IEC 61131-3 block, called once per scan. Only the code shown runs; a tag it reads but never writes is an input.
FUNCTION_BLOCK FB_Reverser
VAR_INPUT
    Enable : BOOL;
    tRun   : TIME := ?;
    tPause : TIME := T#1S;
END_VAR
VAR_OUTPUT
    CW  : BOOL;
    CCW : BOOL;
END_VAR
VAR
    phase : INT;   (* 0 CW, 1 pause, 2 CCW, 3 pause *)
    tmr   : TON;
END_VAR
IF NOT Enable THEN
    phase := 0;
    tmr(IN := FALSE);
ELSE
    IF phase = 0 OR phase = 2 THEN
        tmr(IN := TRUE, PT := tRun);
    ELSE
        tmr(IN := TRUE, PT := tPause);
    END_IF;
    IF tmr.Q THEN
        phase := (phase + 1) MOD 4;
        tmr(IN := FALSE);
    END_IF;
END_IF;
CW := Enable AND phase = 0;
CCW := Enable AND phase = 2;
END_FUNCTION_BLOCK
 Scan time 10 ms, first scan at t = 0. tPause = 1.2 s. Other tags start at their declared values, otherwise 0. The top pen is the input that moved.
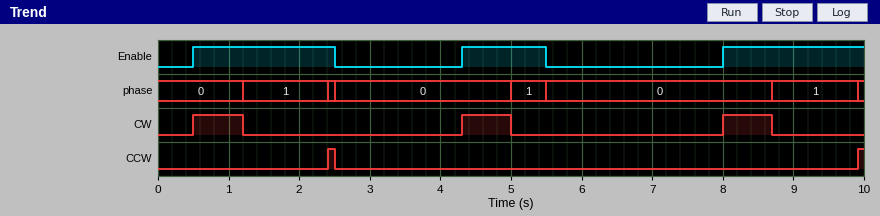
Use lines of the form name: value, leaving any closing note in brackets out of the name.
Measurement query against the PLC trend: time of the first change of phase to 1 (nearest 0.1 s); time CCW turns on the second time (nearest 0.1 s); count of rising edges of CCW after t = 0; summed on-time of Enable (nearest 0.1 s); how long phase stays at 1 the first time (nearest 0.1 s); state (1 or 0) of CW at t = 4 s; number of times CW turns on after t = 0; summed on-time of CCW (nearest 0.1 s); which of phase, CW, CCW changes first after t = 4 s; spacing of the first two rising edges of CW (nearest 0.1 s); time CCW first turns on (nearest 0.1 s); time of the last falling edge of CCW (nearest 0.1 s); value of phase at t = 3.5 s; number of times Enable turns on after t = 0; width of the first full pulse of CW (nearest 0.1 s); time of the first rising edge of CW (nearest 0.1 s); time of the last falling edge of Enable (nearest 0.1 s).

time of the first change of phase to 1: 1.2 s
time CCW turns on the second time: 9.9 s
count of rising edges of CCW after t = 0: 2
summed on-time of Enable: 5.2 s
how long phase stays at 1 the first time: 1.2 s
state (1 or 0) of CW at t = 4 s: 0
number of times CW turns on after t = 0: 3
summed on-time of CCW: 0.2 s
which of phase, CW, CCW changes first after t = 4 s: CW
spacing of the first two rising edges of CW: 3.8 s
time CCW first turns on: 2.4 s
time of the last falling edge of CCW: 2.5 s
value of phase at t = 3.5 s: 0
number of times Enable turns on after t = 0: 3
width of the first full pulse of CW: 0.7 s
time of the first rising edge of CW: 0.5 s
time of the last falling edge of Enable: 5.5 s
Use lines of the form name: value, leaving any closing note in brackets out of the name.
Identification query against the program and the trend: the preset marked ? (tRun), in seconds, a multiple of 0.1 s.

the preset marked ? (tRun), in seconds, a multiple of 0.1 s: 0.7 s
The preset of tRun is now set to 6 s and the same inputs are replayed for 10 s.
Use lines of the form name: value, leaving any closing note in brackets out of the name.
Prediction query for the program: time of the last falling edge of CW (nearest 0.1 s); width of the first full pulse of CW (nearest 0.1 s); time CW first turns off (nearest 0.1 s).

time of the last falling edge of CW: 5.5 s
width of the first full pulse of CW: 2.0 s
time CW first turns off: 2.5 s
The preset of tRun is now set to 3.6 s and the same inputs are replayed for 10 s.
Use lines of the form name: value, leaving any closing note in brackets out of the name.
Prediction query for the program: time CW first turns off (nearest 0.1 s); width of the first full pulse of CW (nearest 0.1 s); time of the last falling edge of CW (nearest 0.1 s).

time CW first turns off: 2.5 s
width of the first full pulse of CW: 2.0 s
time of the last falling edge of CW: 5.5 s
